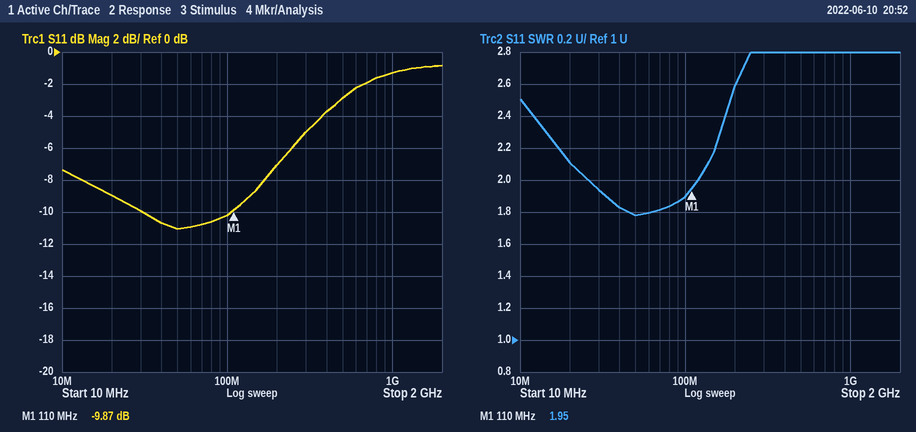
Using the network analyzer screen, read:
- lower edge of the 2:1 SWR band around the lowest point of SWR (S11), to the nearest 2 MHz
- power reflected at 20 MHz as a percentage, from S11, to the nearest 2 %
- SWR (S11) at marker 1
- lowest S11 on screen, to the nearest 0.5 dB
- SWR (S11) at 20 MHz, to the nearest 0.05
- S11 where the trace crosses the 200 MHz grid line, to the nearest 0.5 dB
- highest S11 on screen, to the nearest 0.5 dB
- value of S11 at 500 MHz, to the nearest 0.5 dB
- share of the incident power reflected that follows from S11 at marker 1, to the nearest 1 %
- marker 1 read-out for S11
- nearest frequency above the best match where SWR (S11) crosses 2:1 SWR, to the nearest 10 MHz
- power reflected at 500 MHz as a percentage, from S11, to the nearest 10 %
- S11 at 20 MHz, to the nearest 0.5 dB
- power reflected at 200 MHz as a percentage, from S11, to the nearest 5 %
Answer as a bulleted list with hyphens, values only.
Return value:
- 26 MHz
- 12 %
- 1.95
- -11.0 dB
- 2.10
- -7.0 dB
- -1.0 dB
- -3.0 dB
- 10 %
- -9.87 dB
- 120 MHz
- 50 %
- -9.0 dB
- 20 %
